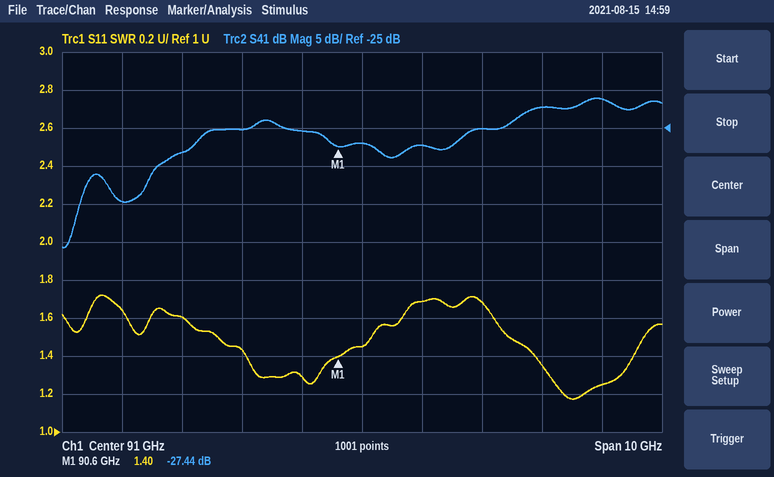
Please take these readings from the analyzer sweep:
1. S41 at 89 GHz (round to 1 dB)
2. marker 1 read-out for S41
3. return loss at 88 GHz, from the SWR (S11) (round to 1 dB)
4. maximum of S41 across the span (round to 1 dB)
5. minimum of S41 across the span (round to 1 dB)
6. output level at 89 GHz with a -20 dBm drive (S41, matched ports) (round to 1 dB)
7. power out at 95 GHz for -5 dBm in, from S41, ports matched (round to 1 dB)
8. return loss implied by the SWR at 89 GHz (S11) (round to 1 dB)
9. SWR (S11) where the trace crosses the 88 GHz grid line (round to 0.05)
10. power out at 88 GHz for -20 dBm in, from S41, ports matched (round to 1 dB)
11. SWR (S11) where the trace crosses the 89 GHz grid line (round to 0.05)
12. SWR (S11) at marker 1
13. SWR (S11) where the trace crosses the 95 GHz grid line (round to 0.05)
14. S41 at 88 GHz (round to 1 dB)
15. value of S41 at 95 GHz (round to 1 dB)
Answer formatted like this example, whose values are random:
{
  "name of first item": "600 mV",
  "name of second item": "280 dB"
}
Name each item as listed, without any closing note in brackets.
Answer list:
{
  "S41 at 89 GHz": "-25 dB",
  "marker 1 read-out for S41": "-27.44 dB",
  "return loss at 88 GHz, from the SWR (S11)": "13 dB",
  "maximum of S41 across the span": "-21 dB",
  "minimum of S41 across the span": "-41 dB",
  "output level at 89 GHz with a -20 dBm drive (S41, matched ports)": "-45 dBm",
  "power out at 95 GHz for -5 dBm in, from S41, ports matched": "-26 dBm",
  "return loss implied by the SWR at 89 GHz (S11)": "15 dB",
  "SWR (S11) where the trace crosses the 88 GHz grid line": "1.60",
  "power out at 88 GHz for -20 dBm in, from S41, ports matched": "-48 dBm",
  "SWR (S11) where the trace crosses the 89 GHz grid line": "1.45",
  "SWR (S11) at marker 1": "1.40",
  "SWR (S11) where the trace crosses the 95 GHz grid line": "1.25",
  "S41 at 88 GHz": "-28 dB",
  "value of S41 at 95 GHz": "-21 dB"
}
